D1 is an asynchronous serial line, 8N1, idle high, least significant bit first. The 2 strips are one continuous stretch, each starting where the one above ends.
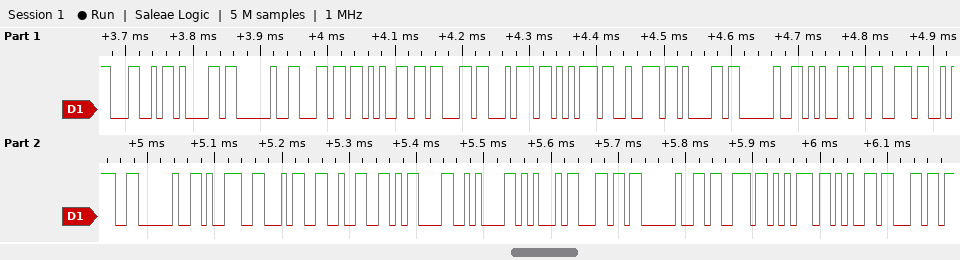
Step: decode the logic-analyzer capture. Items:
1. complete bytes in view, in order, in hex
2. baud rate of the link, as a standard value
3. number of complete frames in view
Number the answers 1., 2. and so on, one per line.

1. 4C 61 20 6C 65 63 74 75 72 61 20 65 73 3A 20 39 34 32 0D 0A 45 6C 20 73 75 65 6C
2. 115200 baud
3. 27
